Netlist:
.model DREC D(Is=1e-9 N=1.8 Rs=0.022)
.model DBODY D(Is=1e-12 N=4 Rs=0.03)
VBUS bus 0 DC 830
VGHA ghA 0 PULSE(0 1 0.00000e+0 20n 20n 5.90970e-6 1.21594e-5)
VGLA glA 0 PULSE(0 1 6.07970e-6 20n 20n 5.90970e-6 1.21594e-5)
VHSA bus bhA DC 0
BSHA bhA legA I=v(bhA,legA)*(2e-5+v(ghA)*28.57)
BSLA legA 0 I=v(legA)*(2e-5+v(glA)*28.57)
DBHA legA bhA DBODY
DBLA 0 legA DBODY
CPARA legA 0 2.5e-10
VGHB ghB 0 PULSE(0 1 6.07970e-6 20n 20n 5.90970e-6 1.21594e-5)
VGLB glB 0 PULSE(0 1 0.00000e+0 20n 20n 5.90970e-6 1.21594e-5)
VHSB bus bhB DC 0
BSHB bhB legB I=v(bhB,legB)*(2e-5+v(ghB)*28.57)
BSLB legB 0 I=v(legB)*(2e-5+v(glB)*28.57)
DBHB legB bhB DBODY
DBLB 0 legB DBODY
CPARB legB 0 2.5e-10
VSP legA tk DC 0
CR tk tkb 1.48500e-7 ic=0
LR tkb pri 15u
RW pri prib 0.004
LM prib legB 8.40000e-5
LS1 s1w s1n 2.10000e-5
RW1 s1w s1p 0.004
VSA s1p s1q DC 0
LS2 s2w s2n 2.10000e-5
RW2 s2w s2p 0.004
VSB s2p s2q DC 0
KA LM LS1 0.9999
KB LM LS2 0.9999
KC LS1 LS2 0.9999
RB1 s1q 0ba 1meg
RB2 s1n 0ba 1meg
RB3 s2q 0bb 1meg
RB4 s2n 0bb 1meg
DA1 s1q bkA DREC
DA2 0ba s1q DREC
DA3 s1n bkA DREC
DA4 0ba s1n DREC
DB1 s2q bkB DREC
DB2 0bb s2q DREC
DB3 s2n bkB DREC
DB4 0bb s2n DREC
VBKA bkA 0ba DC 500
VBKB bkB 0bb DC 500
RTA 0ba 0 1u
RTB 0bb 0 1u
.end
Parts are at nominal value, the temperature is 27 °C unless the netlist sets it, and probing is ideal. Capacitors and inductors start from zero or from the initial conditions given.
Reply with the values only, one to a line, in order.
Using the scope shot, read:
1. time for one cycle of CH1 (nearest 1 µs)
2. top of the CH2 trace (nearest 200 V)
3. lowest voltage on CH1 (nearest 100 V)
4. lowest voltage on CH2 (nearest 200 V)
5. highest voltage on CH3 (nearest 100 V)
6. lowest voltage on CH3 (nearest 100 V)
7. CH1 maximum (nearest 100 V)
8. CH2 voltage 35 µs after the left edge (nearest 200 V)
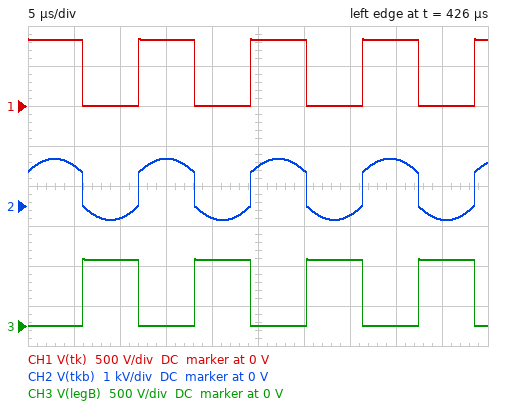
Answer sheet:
12 µs
1.2 kV
0 V
-400 V
800 V
0 V
800 V
-200 V
